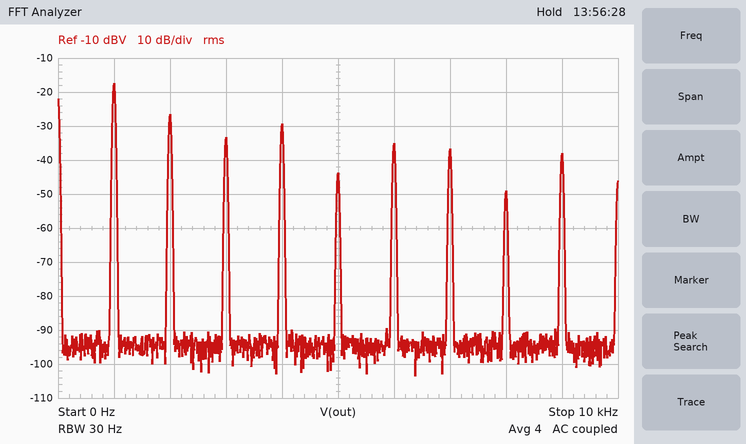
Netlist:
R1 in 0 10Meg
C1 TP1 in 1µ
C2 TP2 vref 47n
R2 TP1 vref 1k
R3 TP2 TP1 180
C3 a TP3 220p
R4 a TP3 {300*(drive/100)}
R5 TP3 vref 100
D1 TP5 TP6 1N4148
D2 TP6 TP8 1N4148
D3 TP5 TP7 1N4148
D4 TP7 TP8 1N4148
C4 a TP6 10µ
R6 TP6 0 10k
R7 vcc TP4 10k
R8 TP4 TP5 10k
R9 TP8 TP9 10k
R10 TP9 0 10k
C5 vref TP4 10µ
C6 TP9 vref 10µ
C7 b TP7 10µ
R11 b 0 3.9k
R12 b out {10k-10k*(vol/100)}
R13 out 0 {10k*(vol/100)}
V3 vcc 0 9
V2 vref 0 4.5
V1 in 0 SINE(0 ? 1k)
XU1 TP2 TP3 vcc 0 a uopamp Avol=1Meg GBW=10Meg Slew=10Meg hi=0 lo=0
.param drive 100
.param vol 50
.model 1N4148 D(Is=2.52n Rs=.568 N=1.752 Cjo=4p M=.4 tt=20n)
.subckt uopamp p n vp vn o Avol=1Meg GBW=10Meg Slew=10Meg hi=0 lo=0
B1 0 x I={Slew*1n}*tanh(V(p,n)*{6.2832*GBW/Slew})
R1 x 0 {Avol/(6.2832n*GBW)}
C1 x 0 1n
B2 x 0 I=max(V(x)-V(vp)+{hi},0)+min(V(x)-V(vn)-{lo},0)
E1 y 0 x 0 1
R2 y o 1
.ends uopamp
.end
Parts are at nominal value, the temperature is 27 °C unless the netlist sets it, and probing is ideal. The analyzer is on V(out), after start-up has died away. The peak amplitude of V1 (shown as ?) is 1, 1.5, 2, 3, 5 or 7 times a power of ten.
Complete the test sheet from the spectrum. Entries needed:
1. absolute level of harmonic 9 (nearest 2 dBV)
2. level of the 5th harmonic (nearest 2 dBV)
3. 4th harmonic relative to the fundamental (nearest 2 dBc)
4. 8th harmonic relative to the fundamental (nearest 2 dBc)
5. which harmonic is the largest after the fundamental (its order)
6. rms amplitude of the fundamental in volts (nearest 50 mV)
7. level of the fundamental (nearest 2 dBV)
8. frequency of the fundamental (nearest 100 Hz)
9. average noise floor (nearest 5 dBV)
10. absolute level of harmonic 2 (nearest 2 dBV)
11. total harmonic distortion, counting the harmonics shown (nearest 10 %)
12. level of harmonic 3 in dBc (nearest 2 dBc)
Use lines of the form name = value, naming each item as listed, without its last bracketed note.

absolute level of harmonic 9 = -38 dBV
level of the 5th harmonic = -44 dBV
4th harmonic relative to the fundamental = -12 dBc
8th harmonic relative to the fundamental = -32 dBc
which harmonic is the largest after the fundamental = 2
rms amplitude of the fundamental in volts = 150 mV
level of the fundamental = -18 dBV
frequency of the fundamental = 1.0 kHz
average noise floor = -95 dBV
absolute level of harmonic 2 = -26 dBV
total harmonic distortion, counting the harmonics shown = 50 %
level of harmonic 3 in dBc = -16 dBc
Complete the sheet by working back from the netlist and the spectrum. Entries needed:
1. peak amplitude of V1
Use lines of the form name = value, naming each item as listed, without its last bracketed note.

peak amplitude of V1 = 1 V
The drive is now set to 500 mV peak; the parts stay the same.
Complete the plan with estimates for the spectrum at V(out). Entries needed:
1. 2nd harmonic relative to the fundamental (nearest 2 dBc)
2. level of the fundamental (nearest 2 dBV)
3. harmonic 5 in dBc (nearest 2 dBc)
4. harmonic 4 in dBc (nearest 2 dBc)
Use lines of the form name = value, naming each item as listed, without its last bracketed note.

2nd harmonic relative to the fundamental = -6 dBc
level of the fundamental = -16 dBV
harmonic 5 in dBc = -18 dBc
harmonic 4 in dBc = -14 dBc
